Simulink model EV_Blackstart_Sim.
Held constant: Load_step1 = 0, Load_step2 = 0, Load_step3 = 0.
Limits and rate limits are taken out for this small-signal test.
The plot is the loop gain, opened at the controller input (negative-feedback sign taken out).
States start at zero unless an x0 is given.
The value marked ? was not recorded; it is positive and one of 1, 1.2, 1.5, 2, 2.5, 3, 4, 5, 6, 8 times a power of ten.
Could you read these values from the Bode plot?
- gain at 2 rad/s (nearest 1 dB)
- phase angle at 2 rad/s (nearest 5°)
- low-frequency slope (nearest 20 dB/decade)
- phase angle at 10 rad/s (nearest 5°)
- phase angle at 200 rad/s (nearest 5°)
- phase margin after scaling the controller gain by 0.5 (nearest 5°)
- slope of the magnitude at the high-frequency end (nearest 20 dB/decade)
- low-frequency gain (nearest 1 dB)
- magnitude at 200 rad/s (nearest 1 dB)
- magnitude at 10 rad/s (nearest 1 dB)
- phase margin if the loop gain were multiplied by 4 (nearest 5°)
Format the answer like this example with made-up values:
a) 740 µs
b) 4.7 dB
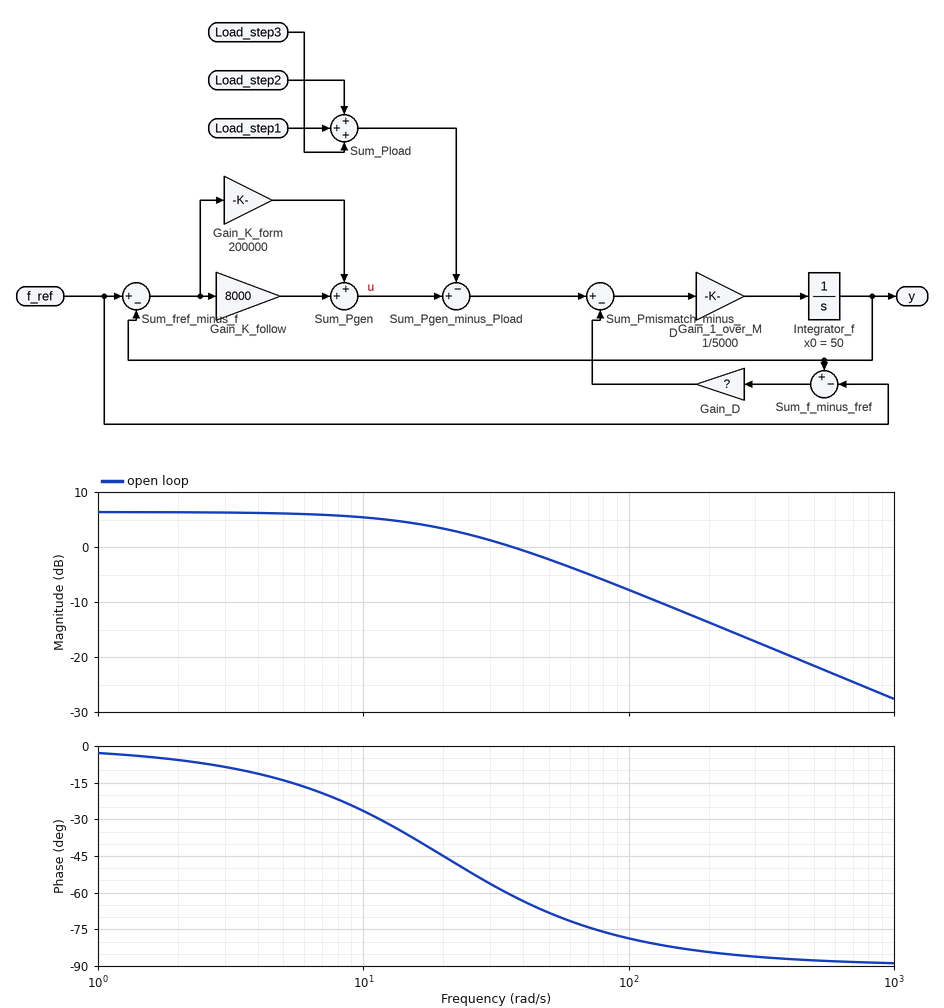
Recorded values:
a) 6 dB
b) -5°
c) 0 dB/decade
d) -25°
e) -85°
f) 165°
g) -20 dB/decade
h) 6 dB
i) -14 dB
j) 5 dB
k) 95°
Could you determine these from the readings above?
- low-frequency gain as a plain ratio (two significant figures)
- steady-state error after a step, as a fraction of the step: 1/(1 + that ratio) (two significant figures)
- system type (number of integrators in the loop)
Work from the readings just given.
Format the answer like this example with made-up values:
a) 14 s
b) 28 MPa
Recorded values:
a) 2.0
b) 0.33
c) 0
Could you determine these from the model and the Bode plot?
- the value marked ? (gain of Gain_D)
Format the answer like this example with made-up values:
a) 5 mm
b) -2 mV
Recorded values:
a) 100000
